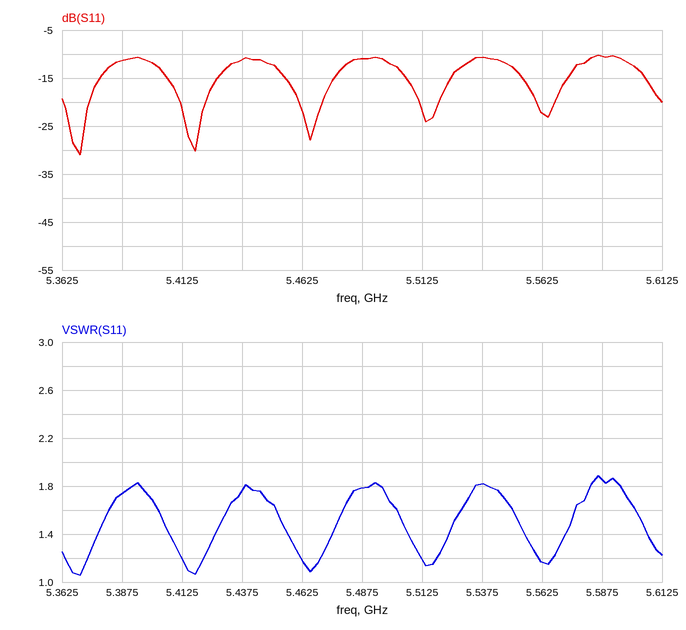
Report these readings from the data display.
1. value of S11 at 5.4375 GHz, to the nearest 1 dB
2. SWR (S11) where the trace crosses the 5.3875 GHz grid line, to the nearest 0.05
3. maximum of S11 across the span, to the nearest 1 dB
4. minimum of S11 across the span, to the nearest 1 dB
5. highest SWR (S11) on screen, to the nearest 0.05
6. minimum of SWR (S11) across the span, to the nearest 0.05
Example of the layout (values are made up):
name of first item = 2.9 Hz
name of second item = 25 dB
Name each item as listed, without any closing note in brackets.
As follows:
value of S11 at 5.4375 GHz, to the nearest 1 dB = -11 dB
SWR (S11) where the trace crosses the 5.3875 GHz grid line, to the nearest 0.05 = 1.75
maximum of S11 across the span, to the nearest 1 dB = -10 dB
minimum of S11 across the span, to the nearest 1 dB = -31 dB
highest SWR (S11) on screen, to the nearest 0.05 = 1.90
minimum of SWR (S11) across the span, to the nearest 0.05 = 1.05
